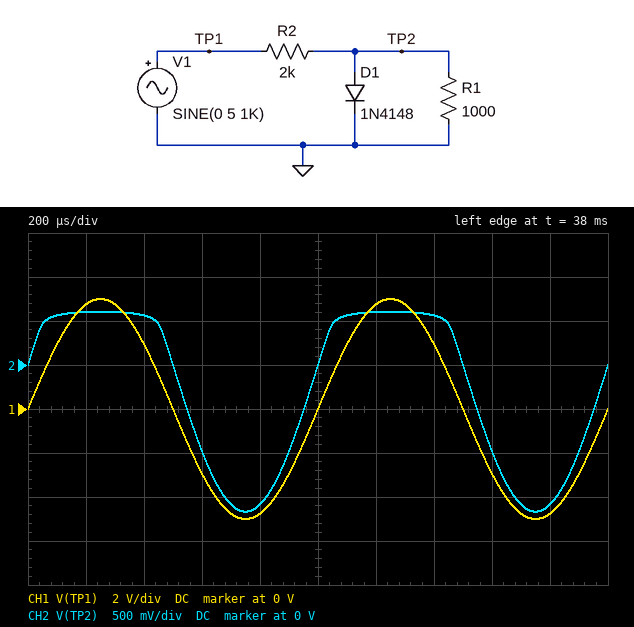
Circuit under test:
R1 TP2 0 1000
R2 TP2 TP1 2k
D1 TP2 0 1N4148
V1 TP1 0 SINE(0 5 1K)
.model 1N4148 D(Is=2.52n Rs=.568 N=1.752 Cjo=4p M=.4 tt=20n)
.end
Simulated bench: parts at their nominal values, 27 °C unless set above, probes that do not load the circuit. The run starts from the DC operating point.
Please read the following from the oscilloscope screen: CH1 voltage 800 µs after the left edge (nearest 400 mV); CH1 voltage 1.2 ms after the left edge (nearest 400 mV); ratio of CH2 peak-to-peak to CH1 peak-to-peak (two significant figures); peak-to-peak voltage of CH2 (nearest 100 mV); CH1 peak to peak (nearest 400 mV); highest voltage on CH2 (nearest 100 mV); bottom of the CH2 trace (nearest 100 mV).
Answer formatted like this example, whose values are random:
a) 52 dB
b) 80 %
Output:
a) -4.8 V
b) 4.8 V
c) 0.23
d) 2.3 V
e) 10.0 V
f) 600 mV
g) -1.7 V
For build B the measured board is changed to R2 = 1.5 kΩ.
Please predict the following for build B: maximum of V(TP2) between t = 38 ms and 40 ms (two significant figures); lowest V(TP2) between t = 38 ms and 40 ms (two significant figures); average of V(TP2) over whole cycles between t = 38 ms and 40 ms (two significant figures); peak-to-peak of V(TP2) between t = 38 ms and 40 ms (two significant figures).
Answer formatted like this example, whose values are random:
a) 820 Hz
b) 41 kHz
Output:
a) 620 mV
b) -2.0 V
c) -370 mV
d) 2.6 V
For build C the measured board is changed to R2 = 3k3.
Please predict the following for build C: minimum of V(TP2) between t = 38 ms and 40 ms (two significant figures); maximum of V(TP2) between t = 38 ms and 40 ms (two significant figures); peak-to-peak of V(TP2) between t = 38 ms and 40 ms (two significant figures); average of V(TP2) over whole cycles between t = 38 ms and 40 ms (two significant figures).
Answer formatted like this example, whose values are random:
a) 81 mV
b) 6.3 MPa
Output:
a) -1.2 V
b) 570 mV
c) 1.7 V
d) -140 mV
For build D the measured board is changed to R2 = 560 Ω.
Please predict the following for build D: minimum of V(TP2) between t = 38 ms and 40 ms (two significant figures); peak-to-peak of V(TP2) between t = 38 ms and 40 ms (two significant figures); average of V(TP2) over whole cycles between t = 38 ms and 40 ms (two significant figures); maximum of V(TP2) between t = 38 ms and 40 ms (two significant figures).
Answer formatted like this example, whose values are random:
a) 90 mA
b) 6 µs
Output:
a) -3.2 V
b) 3.9 V
c) -720 mV
d) 680 mV
